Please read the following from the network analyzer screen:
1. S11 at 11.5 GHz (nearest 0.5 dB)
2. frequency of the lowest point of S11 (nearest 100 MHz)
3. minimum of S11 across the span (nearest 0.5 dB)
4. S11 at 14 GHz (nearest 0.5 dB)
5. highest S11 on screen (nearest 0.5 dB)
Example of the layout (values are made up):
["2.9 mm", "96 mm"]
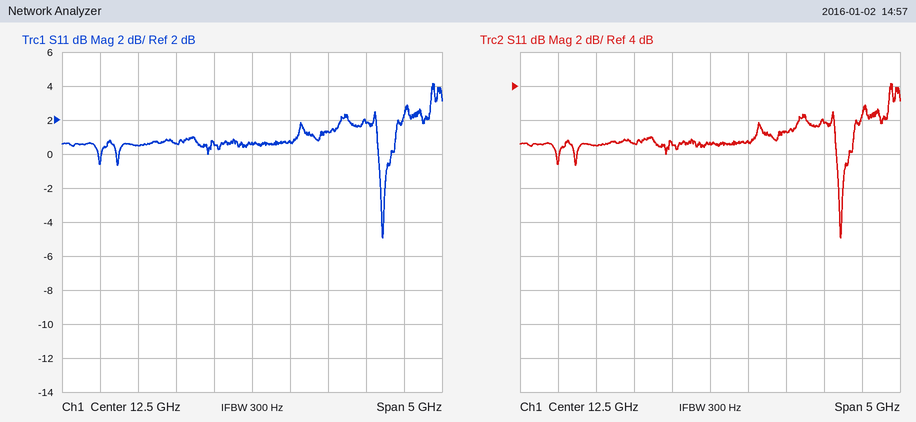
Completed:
["0.5 dB", "14.2 GHz", "-5.0 dB", "2.0 dB", "4.0 dB"]
